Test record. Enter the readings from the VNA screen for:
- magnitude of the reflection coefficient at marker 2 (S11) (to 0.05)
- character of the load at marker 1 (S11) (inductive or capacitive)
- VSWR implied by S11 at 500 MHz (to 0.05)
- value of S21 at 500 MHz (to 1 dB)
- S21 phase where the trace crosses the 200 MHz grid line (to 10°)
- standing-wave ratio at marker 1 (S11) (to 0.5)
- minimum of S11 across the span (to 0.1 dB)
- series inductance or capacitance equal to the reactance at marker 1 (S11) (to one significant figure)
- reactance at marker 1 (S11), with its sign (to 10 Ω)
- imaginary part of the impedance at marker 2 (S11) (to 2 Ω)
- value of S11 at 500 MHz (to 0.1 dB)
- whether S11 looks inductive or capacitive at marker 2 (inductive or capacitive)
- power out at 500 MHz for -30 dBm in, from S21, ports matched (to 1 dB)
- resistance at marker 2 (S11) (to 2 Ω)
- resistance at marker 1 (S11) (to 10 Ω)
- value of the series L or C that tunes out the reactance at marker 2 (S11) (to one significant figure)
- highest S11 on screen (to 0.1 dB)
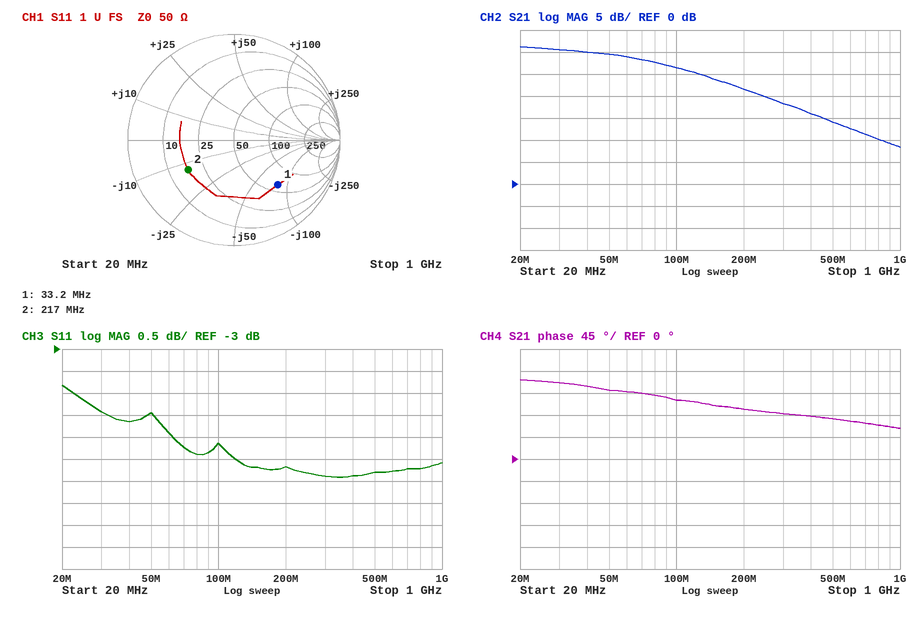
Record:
0.50
capacitive
3.10
14 dB
100°
4.0
-5.9 dB
60 pF
-80 Ω
-14 Ω
-5.8 dB
capacitive
-16 dBm
18 Ω
60 Ω
10 nH
-3.8 dB
